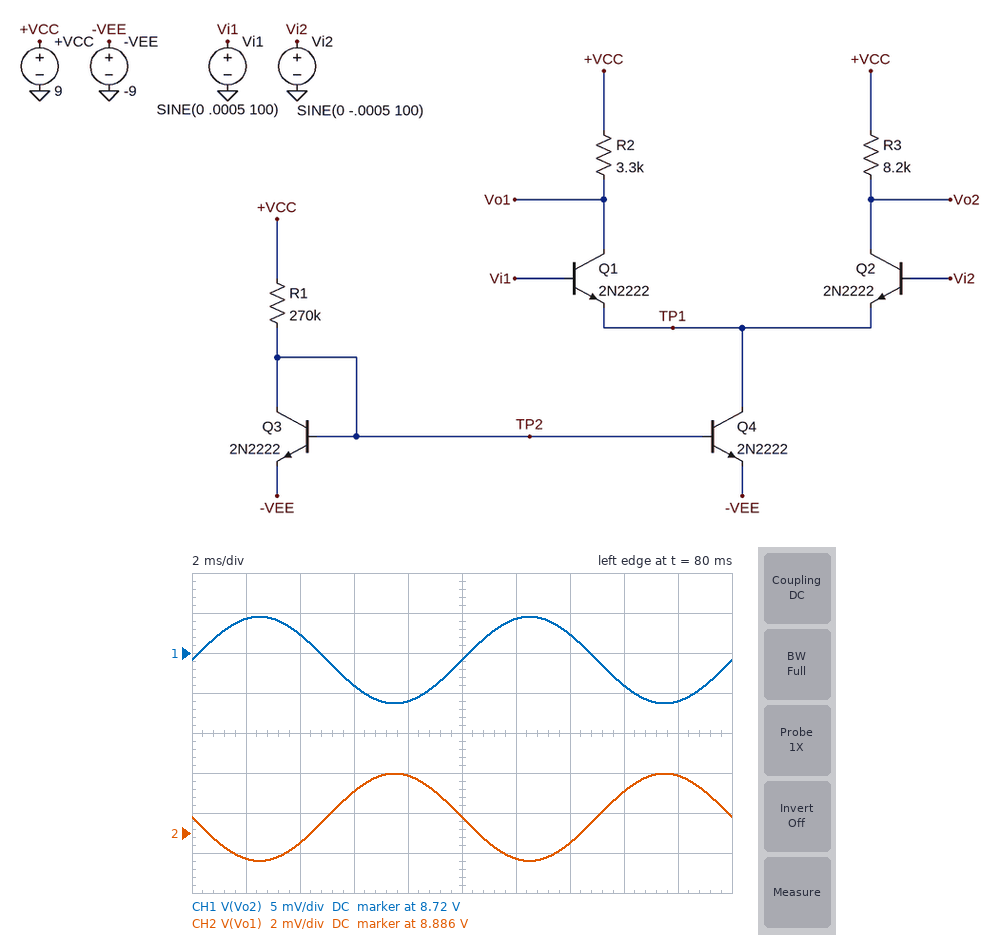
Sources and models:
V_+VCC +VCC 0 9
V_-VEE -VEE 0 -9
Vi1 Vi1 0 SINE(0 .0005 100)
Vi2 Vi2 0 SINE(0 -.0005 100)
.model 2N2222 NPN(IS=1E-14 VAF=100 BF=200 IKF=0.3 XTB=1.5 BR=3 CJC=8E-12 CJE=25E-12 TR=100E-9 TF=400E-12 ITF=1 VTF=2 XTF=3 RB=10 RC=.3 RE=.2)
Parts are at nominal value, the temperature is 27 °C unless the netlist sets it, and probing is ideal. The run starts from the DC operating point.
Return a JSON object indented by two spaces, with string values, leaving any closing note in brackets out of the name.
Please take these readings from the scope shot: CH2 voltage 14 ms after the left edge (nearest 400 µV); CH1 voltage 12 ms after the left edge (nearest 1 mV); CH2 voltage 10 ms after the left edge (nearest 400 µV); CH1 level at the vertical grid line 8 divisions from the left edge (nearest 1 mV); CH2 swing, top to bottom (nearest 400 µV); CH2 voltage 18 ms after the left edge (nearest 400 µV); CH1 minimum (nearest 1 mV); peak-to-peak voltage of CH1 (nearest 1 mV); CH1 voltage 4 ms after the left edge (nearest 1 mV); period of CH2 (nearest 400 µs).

{
  "CH2 voltage 14 ms after the left edge": "8.8856 V",
  "CH1 voltage 12 ms after the left edge": "8.724 V",
  "CH2 voltage 10 ms after the left edge": "8.8868 V",
  "CH1 level at the vertical grid line 8 divisions from the left edge": "8.716 V",
  "CH2 swing, top to bottom": "4.4 mV",
  "CH2 voltage 18 ms after the left edge": "8.8888 V",
  "CH1 minimum": "8.714 V",
  "peak-to-peak voltage of CH1": "11 mV",
  "CH1 voltage 4 ms after the left edge": "8.722 V",
  "period of CH2": "10.0 ms"
}
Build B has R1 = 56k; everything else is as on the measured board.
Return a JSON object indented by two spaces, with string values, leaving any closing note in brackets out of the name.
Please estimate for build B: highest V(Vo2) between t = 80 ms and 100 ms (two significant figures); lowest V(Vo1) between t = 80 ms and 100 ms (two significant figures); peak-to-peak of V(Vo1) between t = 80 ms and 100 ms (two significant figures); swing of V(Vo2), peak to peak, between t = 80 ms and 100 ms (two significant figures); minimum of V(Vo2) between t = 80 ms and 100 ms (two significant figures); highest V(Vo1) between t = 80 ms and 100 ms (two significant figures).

{
  "highest V(Vo2) between t = 80 ms and 100 ms": "7.7 V",
  "lowest V(Vo1) between t = 80 ms and 100 ms": "8.4 V",
  "peak-to-peak of V(Vo1) between t = 80 ms and 100 ms": "21 mV",
  "swing of V(Vo2), peak to peak, between t = 80 ms and 100 ms": "52 mV",
  "minimum of V(Vo2) between t = 80 ms and 100 ms": "7.6 V",
  "highest V(Vo1) between t = 80 ms and 100 ms": "8.5 V"
}
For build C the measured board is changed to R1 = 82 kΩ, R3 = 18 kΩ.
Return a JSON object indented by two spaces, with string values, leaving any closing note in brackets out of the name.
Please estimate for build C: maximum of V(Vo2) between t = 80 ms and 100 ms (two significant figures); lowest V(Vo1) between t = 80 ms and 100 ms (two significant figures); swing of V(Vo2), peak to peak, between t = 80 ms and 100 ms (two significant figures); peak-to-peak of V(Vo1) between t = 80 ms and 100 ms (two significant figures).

{
  "maximum of V(Vo2) between t = 80 ms and 100 ms": "7.0 V",
  "lowest V(Vo1) between t = 80 ms and 100 ms": "8.6 V",
  "swing of V(Vo2), peak to peak, between t = 80 ms and 100 ms": "77 mV",
  "peak-to-peak of V(Vo1) between t = 80 ms and 100 ms": "14 mV"
}
